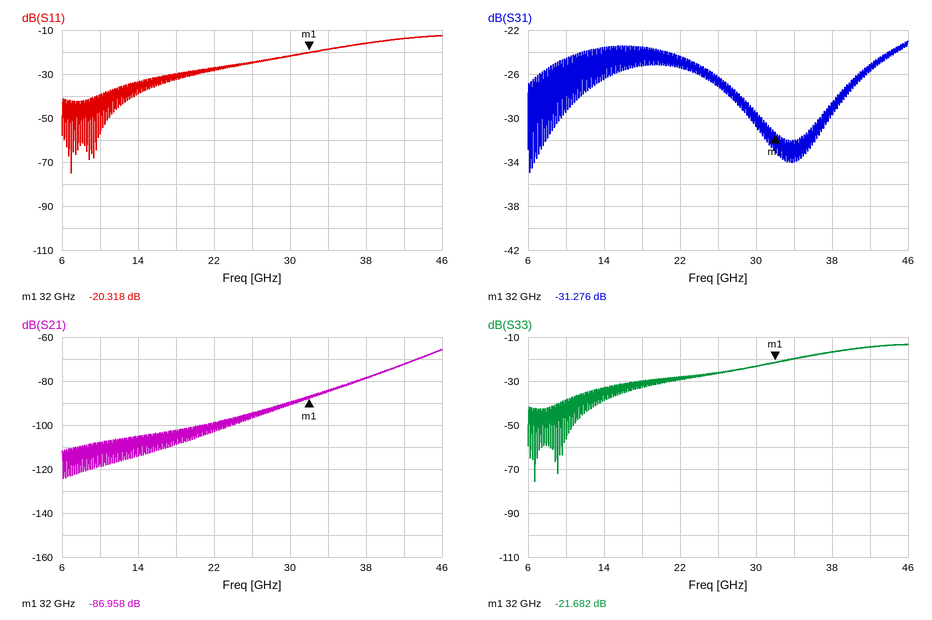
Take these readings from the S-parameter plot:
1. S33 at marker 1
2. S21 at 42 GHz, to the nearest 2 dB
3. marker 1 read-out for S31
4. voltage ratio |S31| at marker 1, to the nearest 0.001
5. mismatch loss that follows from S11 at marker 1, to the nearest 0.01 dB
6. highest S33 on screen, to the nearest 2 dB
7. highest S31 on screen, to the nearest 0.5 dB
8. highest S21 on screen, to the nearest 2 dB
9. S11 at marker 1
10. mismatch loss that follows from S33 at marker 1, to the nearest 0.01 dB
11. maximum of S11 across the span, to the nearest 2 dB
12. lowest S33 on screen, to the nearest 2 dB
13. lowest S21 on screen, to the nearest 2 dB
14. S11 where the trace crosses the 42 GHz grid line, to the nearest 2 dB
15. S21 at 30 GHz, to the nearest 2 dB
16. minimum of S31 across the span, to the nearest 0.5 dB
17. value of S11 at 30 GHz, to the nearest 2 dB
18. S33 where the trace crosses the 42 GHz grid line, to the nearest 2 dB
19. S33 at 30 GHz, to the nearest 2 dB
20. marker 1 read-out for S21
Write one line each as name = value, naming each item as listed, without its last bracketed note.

S33 at marker 1 = -21.682 dB
S21 at 42 GHz, to the nearest 2 dB = -72 dB
marker 1 read-out for S31 = -31.276 dB
voltage ratio |S31| at marker 1, to the nearest 0.001 = 0.027
mismatch loss that follows from S11 at marker 1, to the nearest 0.01 dB = 0.04 dB
highest S33 on screen, to the nearest 2 dB = -14 dB
highest S31 on screen, to the nearest 0.5 dB = -23.0 dB
highest S21 on screen, to the nearest 2 dB = -66 dB
S11 at marker 1 = -20.318 dB
mismatch loss that follows from S33 at marker 1, to the nearest 0.01 dB = 0.03 dB
maximum of S11 across the span, to the nearest 2 dB = -12 dB
lowest S33 on screen, to the nearest 2 dB = -76 dB
lowest S21 on screen, to the nearest 2 dB = -124 dB
S11 where the trace crosses the 42 GHz grid line, to the nearest 2 dB = -14 dB
S21 at 30 GHz, to the nearest 2 dB = -90 dB
minimum of S31 across the span, to the nearest 0.5 dB = -35.0 dB
value of S11 at 30 GHz, to the nearest 2 dB = -22 dB
S33 where the trace crosses the 42 GHz grid line, to the nearest 2 dB = -14 dB
S33 at 30 GHz, to the nearest 2 dB = -24 dB
marker 1 read-out for S21 = -86.958 dB
